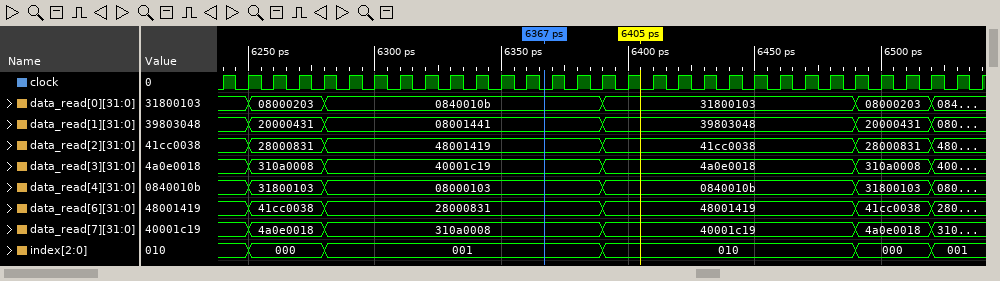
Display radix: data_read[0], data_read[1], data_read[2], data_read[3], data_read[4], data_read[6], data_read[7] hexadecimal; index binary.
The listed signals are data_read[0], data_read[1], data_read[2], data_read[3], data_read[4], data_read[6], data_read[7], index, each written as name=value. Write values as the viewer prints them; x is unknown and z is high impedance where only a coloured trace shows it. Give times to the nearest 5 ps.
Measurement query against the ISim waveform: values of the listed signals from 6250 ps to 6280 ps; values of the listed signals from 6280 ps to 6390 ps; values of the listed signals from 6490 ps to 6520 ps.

data_read[0]=08000203, data_read[1]=20000431, data_read[2]=28000831, data_read[3]=310a0008, data_read[4]=31800103, data_read[6]=41cc0038, data_read[7]=4a0e0018, index=000
data_read[0]=0840010b, data_read[1]=08001441, data_read[2]=48001419, data_read[3]=40001c19, data_read[4]=08000103, data_read[6]=28000831, data_read[7]=310a0008, index=001
data_read[0]=08000203, data_read[1]=20000431, data_read[2]=28000831, data_read[3]=310a0008, data_read[4]=31800103, data_read[6]=41cc0038, data_read[7]=4a0e0018, index=000
